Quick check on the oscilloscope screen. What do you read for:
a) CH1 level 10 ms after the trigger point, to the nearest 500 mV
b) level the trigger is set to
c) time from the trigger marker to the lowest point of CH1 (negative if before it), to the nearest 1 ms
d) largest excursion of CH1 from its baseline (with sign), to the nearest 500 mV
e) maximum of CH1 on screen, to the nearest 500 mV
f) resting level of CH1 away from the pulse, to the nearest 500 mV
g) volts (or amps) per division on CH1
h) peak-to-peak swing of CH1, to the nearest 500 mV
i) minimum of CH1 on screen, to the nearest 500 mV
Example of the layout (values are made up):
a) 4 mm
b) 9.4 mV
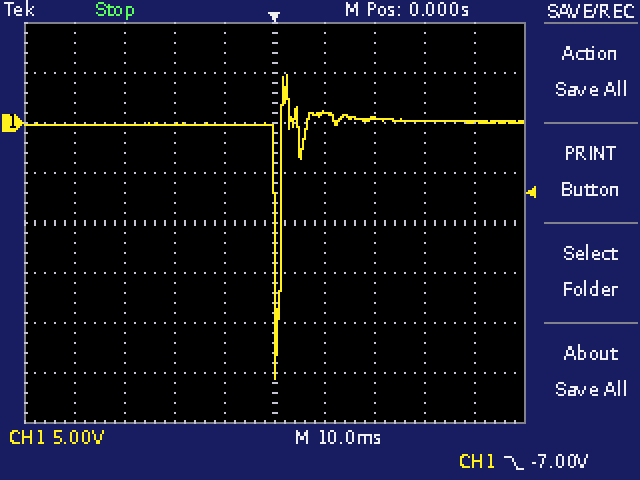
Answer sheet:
a) 1.0 V
b) -7.00 V
c) 0 ms
d) -25.5 V
e) 5.0 V
f) 0.0 V
g) 5 V
h) 30.5 V
i) -25.5 V
